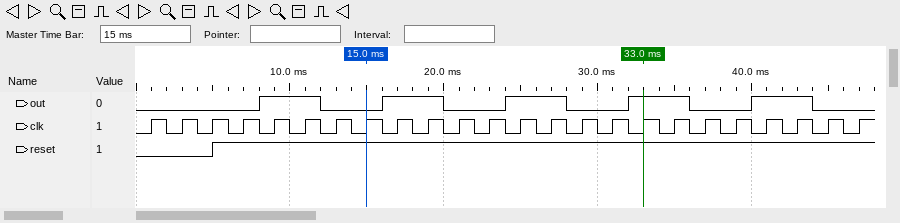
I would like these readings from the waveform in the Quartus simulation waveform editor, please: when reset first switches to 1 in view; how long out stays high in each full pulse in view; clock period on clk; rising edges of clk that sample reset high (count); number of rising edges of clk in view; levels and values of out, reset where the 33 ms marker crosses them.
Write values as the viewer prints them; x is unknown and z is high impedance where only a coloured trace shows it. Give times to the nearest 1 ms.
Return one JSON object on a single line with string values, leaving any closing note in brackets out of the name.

{"when reset first switches to 1 in view": "5 ms", "how long out stays high in each full pulse in view": "4 ms, 4 ms, 4 ms, 4 ms, 4 ms", "clock period on clk": "2 ms", "rising edges of clk that sample reset high": "21", "number of rising edges of clk in view": "24", "levels and values of out, reset where the 33 ms marker crosses them": "out=1, reset=1"}
